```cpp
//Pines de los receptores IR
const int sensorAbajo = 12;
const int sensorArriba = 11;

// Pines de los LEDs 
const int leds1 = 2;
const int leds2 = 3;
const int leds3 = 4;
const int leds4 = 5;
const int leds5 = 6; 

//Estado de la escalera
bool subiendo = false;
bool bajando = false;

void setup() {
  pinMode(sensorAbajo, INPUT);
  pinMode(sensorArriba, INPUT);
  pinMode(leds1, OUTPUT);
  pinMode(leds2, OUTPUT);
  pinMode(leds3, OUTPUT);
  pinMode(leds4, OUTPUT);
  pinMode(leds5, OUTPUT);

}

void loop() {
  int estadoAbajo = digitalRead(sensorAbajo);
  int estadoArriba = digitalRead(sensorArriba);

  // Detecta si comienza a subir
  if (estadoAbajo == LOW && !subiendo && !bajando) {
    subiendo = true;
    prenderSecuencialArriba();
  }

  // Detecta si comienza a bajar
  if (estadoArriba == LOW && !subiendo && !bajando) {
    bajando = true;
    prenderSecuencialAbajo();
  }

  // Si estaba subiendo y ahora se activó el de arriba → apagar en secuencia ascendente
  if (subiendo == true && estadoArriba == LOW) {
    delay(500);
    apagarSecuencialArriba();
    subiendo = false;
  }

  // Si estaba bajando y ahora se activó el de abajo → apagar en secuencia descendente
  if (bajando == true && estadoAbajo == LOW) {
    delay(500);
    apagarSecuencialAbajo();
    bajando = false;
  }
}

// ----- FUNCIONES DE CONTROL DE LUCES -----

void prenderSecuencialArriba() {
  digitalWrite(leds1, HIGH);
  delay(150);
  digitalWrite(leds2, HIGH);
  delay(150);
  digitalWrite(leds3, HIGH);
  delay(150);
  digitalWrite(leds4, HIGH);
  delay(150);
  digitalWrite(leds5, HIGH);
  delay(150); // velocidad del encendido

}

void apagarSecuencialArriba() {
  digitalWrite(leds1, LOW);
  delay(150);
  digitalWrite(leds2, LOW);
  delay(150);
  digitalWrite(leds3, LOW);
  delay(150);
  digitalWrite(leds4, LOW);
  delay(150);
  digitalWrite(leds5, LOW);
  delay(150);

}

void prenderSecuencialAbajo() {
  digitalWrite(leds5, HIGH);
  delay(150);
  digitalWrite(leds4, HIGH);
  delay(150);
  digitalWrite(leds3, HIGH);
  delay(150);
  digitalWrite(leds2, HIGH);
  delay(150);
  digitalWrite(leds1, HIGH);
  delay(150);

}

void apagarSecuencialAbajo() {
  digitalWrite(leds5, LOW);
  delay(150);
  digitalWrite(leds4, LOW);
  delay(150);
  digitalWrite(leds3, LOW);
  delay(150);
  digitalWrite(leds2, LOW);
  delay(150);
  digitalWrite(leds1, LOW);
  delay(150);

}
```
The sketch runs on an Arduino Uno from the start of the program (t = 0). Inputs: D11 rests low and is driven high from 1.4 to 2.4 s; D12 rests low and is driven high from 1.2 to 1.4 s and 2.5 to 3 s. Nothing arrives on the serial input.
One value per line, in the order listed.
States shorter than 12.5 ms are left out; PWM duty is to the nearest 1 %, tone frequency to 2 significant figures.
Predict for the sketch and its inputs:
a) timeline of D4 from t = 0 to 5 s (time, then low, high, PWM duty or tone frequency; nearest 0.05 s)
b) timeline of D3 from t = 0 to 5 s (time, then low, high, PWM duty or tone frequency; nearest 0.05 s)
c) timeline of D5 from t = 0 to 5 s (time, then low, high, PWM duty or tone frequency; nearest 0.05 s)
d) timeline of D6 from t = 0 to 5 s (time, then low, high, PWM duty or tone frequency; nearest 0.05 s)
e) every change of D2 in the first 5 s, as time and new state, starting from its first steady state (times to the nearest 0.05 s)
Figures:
0 s low; 0.3 s high; 1.55 s low; 2.3 s high; 3.55 s low; 4.3 s high
0 s low; 0.15 s high; 1.4 s low; 2.15 s high; 3.4 s low; 4.15 s high
0 s low; 0.45 s high; 1.7 s low; 2.45 s high; 3.7 s low; 4.45 s high
0 s low; 0.6 s high; 1.85 s low; 2.6 s high; 3.85 s low; 4.6 s high
0 s high; 1.25 s low; 2 s high; 3.25 s low; 4 s high
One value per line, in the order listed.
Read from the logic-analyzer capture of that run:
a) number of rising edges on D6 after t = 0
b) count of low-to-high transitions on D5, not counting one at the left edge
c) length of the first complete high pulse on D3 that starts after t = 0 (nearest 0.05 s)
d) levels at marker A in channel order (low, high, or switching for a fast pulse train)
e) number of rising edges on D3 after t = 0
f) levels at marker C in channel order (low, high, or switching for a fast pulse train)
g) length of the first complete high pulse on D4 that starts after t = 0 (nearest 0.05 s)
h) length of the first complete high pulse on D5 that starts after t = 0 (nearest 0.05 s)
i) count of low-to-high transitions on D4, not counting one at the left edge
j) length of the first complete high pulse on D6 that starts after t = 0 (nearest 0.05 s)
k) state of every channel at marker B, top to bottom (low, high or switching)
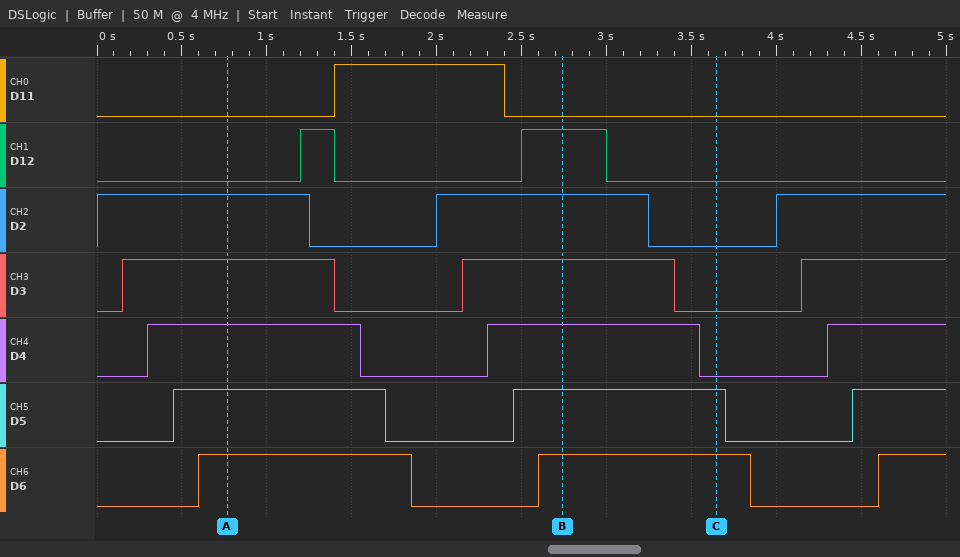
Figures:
3
3
1.25 s
D11 low, D12 low, D2 high, D3 high, D4 high, D5 high, D6 high
3
D11 low, D12 low, D2 low, D3 low, D4 low, D5 high, D6 high
1.25 s
1.25 s
3
1.25 s
D11 low, D12 high, D2 high, D3 high, D4 high, D5 high, D6 high
